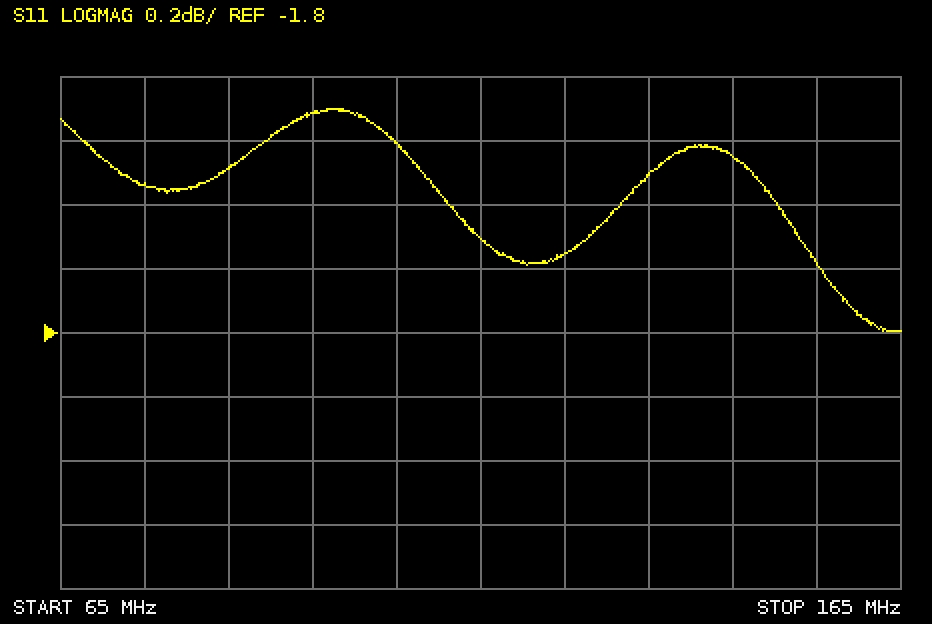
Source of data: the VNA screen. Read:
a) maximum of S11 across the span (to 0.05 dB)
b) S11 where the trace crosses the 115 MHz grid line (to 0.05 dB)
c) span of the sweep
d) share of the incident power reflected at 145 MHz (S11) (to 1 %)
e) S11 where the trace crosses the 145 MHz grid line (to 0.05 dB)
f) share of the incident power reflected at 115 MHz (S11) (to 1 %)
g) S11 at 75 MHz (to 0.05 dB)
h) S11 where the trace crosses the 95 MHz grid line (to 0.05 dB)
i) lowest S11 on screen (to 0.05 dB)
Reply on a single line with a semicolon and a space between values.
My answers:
-1.10 dB; -1.50 dB; 100 MHz; 75 %; -1.25 dB; 71 %; -1.35 dB; -1.10 dB; -1.80 dB
